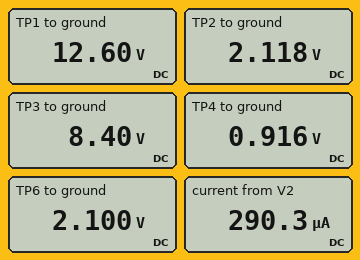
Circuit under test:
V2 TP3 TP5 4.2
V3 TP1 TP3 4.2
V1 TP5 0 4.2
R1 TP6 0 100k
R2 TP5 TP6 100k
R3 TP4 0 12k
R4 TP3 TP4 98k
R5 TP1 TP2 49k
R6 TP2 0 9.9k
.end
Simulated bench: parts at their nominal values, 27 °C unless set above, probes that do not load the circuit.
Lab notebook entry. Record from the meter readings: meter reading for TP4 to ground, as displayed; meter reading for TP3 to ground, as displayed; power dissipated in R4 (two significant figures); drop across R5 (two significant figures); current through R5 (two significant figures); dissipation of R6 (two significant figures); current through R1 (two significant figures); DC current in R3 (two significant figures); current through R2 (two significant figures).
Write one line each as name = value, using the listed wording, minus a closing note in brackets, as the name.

meter reading for TP4 to ground, as displayed = 0.916 V
meter reading for TP3 to ground, as displayed = 8.40 V
power dissipated in R4 = 570 µW
drop across R5 = 10 V
current through R5 = 210 µA
dissipation of R6 = 450 µW
current through R1 = 21 µA
DC current in R3 = 76 µA
current through R2 = 21 µA
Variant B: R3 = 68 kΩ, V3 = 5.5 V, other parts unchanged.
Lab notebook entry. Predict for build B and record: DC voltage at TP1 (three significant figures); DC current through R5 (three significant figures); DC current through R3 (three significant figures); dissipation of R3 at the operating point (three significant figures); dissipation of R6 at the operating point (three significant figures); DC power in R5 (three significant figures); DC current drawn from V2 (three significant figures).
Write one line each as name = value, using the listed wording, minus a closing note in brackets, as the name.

DC voltage at TP1 = 13.9 V
DC current through R5 = 236 µA
DC current through R3 = 50.6 µA
dissipation of R3 at the operating point = 174 µW
dissipation of R6 at the operating point = 551 µW
DC power in R5 = 2.73 mW
DC current drawn from V2 = 287 µA
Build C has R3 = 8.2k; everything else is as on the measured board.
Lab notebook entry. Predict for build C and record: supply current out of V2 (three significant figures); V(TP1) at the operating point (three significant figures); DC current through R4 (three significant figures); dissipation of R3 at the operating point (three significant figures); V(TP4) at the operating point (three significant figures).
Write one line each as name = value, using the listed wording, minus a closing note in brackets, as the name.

supply current out of V2 = 293 µA
V(TP1) at the operating point = 12.6 V
DC current through R4 = 79.1 µA
dissipation of R3 at the operating point = 51.3 µW
V(TP4) at the operating point = 649 mV
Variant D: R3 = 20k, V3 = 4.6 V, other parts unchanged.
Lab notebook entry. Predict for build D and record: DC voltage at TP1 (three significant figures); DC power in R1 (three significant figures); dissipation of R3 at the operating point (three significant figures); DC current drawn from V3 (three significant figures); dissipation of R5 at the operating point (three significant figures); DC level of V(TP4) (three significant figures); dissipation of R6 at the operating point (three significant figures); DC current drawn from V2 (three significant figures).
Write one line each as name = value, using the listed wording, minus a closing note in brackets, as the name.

DC voltage at TP1 = 13.0 V
DC power in R1 = 44.1 µW
dissipation of R3 at the operating point = 101 µW
DC current drawn from V3 = 221 µA
dissipation of R5 at the operating point = 2.39 mW
DC level of V(TP4) = 1.42 V
dissipation of R6 at the operating point = 482 µW
DC current drawn from V2 = 292 µA
